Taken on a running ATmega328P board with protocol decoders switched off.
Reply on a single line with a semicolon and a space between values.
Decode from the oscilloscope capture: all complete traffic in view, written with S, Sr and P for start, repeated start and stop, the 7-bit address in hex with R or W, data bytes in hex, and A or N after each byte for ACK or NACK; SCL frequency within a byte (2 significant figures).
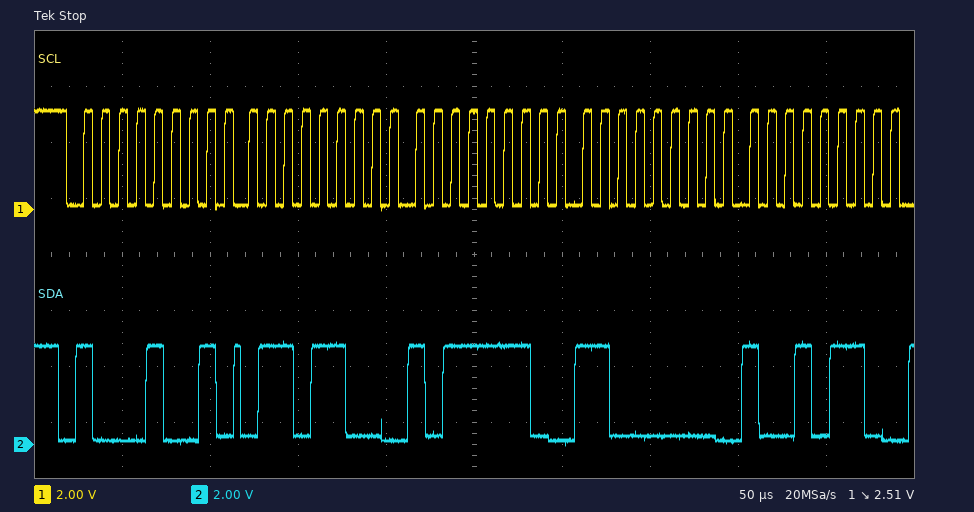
S 44R A 6C A BE A C0 A 96 A; 100 kHz
